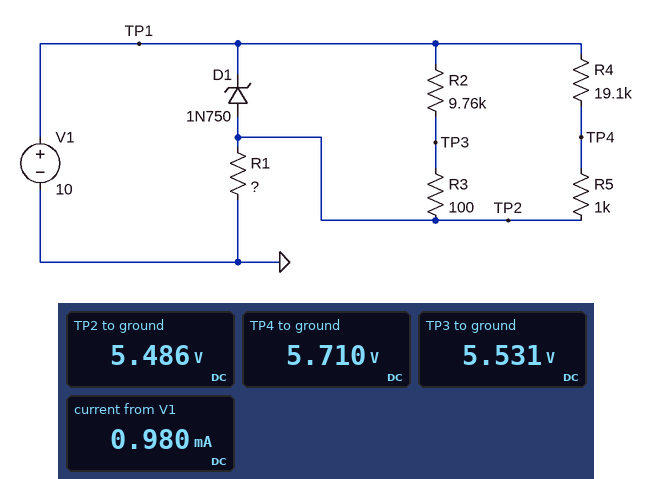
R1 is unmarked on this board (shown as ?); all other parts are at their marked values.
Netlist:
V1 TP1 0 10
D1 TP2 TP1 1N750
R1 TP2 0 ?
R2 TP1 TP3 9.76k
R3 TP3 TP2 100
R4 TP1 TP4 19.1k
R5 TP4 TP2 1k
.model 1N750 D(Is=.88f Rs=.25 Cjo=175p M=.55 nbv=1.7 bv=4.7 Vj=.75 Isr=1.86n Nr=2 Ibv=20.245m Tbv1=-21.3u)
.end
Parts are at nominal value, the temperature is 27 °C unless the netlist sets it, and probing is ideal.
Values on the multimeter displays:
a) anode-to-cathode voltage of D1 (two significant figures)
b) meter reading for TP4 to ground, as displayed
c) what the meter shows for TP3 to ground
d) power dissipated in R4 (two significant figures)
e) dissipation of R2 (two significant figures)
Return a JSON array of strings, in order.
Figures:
["-4.5 V", "5.710 V", "5.531 V", "960 µW", "2.0 mW"]
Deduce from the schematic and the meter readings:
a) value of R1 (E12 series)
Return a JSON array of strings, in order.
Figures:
["5.6 kΩ"]
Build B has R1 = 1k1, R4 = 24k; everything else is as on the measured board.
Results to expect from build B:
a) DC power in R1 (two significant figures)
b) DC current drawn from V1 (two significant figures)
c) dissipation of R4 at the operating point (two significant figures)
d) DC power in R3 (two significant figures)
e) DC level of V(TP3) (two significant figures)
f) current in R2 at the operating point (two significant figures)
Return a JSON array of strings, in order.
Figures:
["26 mW", "4.9 mA", "820 µW", "22 µW", "5.4 V", "470 µA"]
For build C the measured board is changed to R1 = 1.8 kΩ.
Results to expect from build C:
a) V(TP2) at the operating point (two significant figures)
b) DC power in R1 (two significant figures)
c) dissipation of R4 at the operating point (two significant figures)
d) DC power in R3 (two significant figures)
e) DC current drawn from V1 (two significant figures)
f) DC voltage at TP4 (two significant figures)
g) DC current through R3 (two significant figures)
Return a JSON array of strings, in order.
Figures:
["5.4 V", "16 mW", "1.0 mW", "22 µW", "3.0 mA", "5.6 V", "470 µA"]
